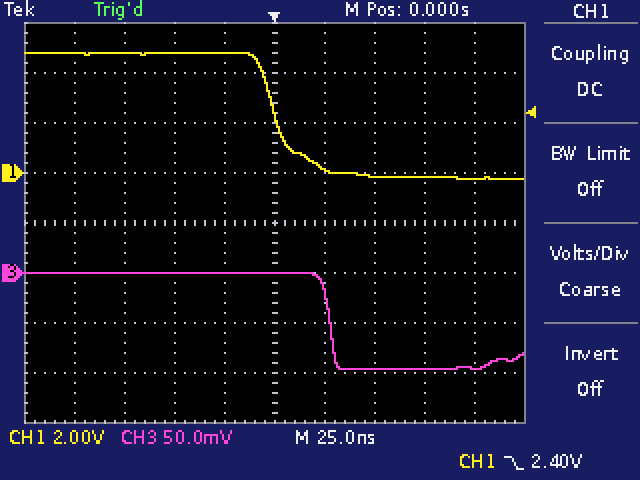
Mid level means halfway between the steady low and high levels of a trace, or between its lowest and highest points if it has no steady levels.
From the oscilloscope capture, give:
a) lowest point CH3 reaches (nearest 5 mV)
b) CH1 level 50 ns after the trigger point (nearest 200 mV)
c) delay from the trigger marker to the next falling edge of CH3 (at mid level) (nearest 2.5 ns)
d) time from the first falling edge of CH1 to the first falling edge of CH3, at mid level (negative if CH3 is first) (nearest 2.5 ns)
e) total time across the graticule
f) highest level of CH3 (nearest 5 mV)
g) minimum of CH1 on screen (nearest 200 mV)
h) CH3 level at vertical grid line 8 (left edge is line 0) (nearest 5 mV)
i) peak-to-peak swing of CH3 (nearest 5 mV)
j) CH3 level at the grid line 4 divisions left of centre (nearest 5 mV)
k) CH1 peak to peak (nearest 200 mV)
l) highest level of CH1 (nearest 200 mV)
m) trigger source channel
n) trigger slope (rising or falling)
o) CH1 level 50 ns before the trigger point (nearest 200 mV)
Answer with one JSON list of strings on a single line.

["-95 mV", "-200 mV", "27.5 ns", "+27.5 ns", "250 ns", "0 mV", "-200 mV", "-95 mV", "95 mV", "0 mV", "5.0 V", "4.8 V", "CH1", "falling", "4.8 V"]
